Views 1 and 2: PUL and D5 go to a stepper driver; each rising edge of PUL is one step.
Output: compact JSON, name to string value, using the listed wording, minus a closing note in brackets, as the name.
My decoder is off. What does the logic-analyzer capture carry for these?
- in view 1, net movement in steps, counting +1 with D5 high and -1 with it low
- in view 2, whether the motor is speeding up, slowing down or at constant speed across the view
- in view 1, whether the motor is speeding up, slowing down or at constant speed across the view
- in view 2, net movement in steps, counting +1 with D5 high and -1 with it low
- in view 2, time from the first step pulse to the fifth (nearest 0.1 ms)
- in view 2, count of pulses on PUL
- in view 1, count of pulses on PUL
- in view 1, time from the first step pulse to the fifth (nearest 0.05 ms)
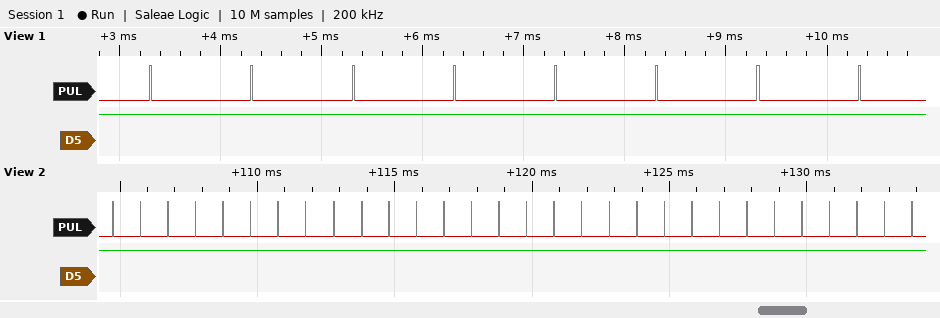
{"in view 1, net movement in steps, counting +1 with D5 high and -1 with it low": "+8", "in view 2, whether the motor is speeding up, slowing down or at constant speed across the view": "constant speed", "in view 1, whether the motor is speeding up, slowing down or at constant speed across the view": "constant speed", "in view 2, net movement in steps, counting +1 with D5 high and -1 with it low": "+30", "in view 2, time from the first step pulse to the fifth": "4.0 ms", "in view 2, count of pulses on PUL": "30", "in view 1, count of pulses on PUL": "8", "in view 1, time from the first step pulse to the fifth": "4.00 ms"}
